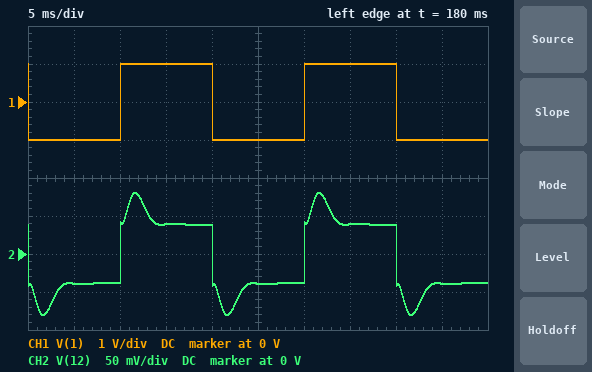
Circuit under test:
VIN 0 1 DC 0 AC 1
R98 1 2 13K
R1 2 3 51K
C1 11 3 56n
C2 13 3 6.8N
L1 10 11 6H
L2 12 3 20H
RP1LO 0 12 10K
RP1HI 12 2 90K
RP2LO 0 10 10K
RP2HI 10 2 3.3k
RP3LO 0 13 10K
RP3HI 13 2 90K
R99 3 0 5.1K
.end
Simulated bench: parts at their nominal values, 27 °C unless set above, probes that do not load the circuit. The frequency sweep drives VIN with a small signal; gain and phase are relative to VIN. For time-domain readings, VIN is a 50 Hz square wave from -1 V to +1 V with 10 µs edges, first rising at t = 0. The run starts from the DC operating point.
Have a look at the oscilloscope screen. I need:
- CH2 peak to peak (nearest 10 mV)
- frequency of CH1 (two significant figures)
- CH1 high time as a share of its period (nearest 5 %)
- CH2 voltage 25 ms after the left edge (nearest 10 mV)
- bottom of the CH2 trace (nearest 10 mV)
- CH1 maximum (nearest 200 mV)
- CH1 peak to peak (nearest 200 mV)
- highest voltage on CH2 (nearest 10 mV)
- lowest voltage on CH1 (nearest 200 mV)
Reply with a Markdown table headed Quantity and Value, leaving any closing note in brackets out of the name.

| Quantity | Value |
|---|---|
| CH2 peak to peak | 160 mV |
| frequency of CH1 | 50 Hz |
| CH1 high time as a share of its period | 50 % |
| CH2 voltage 25 ms after the left edge | -40 mV |
| bottom of the CH2 trace | -80 mV |
| CH1 maximum | 1.0 V |
| CH1 peak to peak | 2.0 V |
| highest voltage on CH2 | 80 mV |
| lowest voltage on CH1 | -1.0 V |
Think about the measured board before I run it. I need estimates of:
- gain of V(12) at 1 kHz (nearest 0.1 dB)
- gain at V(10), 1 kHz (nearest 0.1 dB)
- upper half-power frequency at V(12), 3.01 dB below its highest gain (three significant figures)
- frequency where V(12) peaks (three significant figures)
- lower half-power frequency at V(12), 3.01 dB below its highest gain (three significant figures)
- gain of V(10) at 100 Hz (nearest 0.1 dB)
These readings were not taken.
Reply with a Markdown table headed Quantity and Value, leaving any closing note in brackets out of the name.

| Quantity | Value |
|---|---|
| gain of V(12) at 1 kHz | -28.5 dB |
| gain at V(10), 1 kHz | -10.5 dB |
| upper half-power frequency at V(12), 3.01 dB below its highest gain | 278 Hz |
| frequency where V(12) peaks | 176 Hz |
| lower half-power frequency at V(12), 3.01 dB below its highest gain | 56.2 Hz |
| gain of V(10) at 100 Hz | -10.7 dB |
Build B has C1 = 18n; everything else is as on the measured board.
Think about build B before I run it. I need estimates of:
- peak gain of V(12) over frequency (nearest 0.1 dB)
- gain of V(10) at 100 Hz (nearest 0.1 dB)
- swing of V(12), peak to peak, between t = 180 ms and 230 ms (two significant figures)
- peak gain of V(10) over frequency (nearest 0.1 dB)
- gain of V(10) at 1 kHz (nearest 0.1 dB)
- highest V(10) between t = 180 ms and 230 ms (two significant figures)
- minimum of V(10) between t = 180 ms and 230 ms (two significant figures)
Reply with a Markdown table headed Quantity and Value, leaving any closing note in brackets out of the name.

| Quantity | Value |
|---|---|
| peak gain of V(12) over frequency | -25.6 dB |
| gain of V(10) at 100 Hz | -10.4 dB |
| swing of V(12), peak to peak, between t = 180 ms and 230 ms | 120 mV |
| peak gain of V(10) over frequency | -10.3 dB |
| gain of V(10) at 1 kHz | -10.6 dB |
| highest V(10) between t = 180 ms and 230 ms | 350 mV |
| minimum of V(10) between t = 180 ms and 230 ms | -350 mV |
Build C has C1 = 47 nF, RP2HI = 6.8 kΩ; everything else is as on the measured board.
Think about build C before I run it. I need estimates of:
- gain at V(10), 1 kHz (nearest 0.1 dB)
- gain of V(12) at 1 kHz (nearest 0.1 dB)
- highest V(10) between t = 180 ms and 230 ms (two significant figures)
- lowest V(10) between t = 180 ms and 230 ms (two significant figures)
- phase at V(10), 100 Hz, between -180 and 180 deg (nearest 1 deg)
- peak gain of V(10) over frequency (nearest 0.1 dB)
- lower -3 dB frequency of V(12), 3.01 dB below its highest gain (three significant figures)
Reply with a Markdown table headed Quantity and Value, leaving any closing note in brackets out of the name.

| Quantity | Value |
|---|---|
| gain at V(10), 1 kHz | -11.9 dB |
| gain of V(12) at 1 kHz | -27.6 dB |
| highest V(10) between t = 180 ms and 230 ms | 290 mV |
| lowest V(10) between t = 180 ms and 230 ms | -290 mV |
| phase at V(10), 100 Hz, between -180 and 180 deg | 171 deg |
| peak gain of V(10) over frequency | -11.6 dB |
| lower -3 dB frequency of V(12), 3.01 dB below its highest gain | 38.3 Hz |
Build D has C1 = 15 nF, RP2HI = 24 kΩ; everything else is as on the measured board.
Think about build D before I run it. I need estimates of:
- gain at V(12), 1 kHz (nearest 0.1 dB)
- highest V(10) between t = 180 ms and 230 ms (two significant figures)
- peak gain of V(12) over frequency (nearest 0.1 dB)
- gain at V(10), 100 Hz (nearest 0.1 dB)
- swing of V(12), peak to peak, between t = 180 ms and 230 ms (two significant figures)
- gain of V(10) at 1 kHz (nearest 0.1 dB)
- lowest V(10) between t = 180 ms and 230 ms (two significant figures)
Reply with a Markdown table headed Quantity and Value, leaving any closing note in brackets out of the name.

| Quantity | Value |
|---|---|
| gain at V(12), 1 kHz | -25.7 dB |
| highest V(10) between t = 180 ms and 230 ms | 180 mV |
| peak gain of V(12) over frequency | -24.9 dB |
| gain at V(10), 100 Hz | -16.1 dB |
| swing of V(12), peak to peak, between t = 180 ms and 230 ms | 120 mV |
| gain of V(10) at 1 kHz | -16.6 dB |
| lowest V(10) between t = 180 ms and 230 ms | -180 mV |
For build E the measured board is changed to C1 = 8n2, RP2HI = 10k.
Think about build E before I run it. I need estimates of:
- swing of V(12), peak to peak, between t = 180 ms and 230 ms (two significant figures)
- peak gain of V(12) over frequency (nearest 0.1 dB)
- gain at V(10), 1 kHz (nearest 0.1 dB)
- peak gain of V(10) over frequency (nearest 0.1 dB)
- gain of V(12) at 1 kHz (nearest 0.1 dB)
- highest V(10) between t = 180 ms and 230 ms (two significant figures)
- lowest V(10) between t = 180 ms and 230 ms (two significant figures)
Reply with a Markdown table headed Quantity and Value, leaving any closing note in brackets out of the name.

| Quantity | Value |
|---|---|
| swing of V(12), peak to peak, between t = 180 ms and 230 ms | 110 mV |
| peak gain of V(12) over frequency | -25.9 dB |
| gain at V(10), 1 kHz | -13.5 dB |
| peak gain of V(10) over frequency | -12.6 dB |
| gain of V(12) at 1 kHz | -27.3 dB |
| highest V(10) between t = 180 ms and 230 ms | 270 mV |
| lowest V(10) between t = 180 ms and 230 ms | -270 mV |
